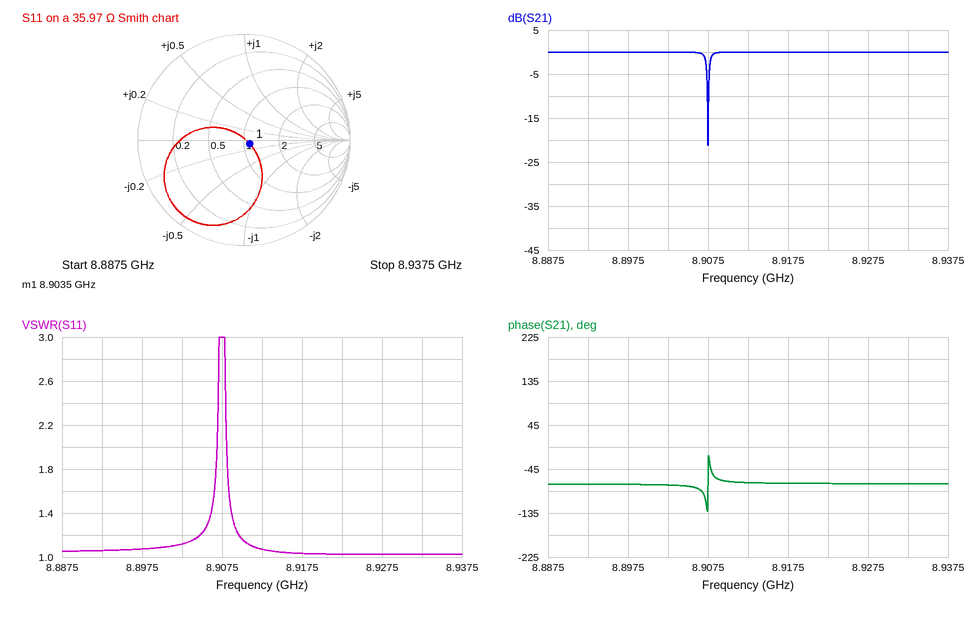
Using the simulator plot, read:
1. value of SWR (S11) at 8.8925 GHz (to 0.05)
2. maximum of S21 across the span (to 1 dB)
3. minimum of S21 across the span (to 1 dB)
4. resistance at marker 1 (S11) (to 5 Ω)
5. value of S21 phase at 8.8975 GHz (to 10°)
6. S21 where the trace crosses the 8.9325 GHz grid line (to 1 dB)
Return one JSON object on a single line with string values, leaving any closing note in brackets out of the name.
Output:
{"value of SWR (S11) at 8.8925 GHz": "1.05", "maximum of S21 across the span": "0 dB", "minimum of S21 across the span": "-21 dB", "resistance at marker 1 (S11)": "40 Ω", "value of S21 phase at 8.8975 GHz": "-80°", "S21 where the trace crosses the 8.9325 GHz grid line": "0 dB"}
